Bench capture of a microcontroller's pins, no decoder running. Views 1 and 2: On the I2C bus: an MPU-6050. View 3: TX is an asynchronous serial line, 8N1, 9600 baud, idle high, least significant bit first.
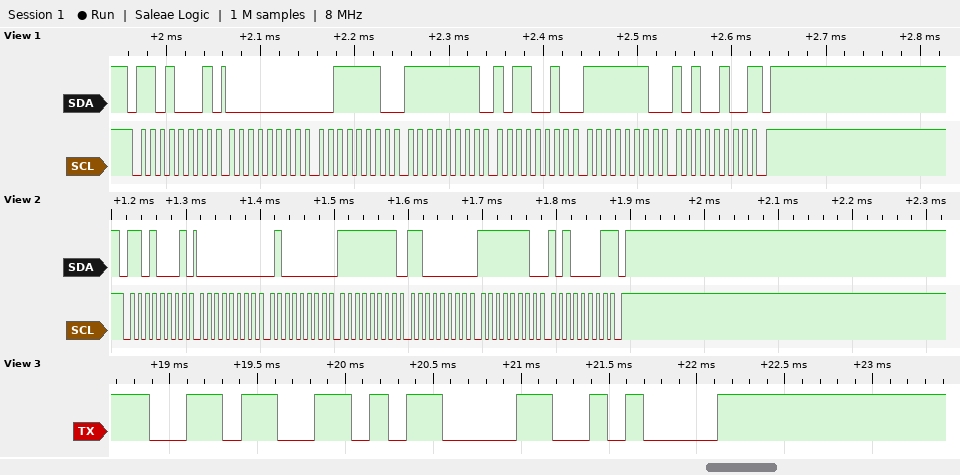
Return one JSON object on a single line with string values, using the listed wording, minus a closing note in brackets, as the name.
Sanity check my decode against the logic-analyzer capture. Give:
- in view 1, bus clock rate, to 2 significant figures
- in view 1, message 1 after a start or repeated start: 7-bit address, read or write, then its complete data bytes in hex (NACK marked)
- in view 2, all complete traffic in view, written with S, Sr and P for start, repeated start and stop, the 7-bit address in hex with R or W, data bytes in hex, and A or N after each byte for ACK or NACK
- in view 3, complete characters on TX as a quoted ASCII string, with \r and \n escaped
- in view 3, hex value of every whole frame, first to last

{"in view 1, bus clock rate, to 2 significant figures": "100 kHz", "in view 1, message 1 after a start or repeated start: 7-bit address, read or write, then its complete data bytes in hex": "0x68 read: 00 3E FF B2 FE A4 NACK", "in view 2, all complete traffic in view, written with S, Sr and P for start, repeated start and stop, the 7-bit address in hex with R or W, data bytes in hex, and A or N after each byte for ACK or NACK": "S 68R A 00 A 40 A FF A C0 A FE A A1 N P", "in view 3, complete characters on TX as a quoted ASCII string, with \\r and \\n escaped": "\"6\\r\\n\"", "in view 3, hex value of every whole frame, first to last": "36 0D 0A"}
